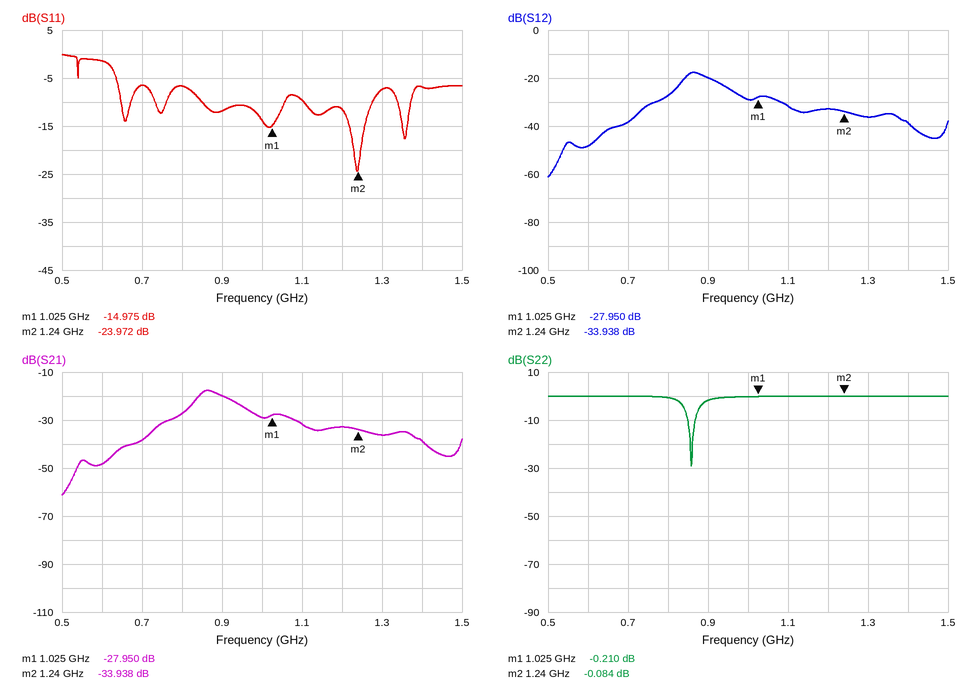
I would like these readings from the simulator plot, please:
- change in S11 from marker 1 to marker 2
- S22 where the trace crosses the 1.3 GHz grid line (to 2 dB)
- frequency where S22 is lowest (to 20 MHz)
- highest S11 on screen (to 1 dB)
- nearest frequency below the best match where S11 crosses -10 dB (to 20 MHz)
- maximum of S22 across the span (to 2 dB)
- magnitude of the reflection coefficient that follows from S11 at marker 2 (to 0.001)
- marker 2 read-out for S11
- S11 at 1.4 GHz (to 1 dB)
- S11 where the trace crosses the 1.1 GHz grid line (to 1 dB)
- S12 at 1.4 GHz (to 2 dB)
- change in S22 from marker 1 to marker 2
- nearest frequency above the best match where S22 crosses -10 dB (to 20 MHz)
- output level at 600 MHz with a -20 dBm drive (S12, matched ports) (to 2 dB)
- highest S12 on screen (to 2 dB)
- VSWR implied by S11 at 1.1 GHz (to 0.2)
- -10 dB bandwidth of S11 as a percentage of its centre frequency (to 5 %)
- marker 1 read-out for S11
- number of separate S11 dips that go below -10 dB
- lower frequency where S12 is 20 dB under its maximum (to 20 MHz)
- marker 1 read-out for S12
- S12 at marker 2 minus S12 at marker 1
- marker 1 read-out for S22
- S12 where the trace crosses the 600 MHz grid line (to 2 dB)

-8.997 dB
0 dB
860 MHz
0 dB
1.10 GHz
0 dB
0.063
-23.972 dB
-7 dB
-10 dB
-38 dB
0.126 dB
860 MHz
-68 dBm
-18 dB
2.0
15 %
-14.975 dB
5
700 MHz
-27.950 dB
-5.988 dB
-0.210 dB
-48 dB
